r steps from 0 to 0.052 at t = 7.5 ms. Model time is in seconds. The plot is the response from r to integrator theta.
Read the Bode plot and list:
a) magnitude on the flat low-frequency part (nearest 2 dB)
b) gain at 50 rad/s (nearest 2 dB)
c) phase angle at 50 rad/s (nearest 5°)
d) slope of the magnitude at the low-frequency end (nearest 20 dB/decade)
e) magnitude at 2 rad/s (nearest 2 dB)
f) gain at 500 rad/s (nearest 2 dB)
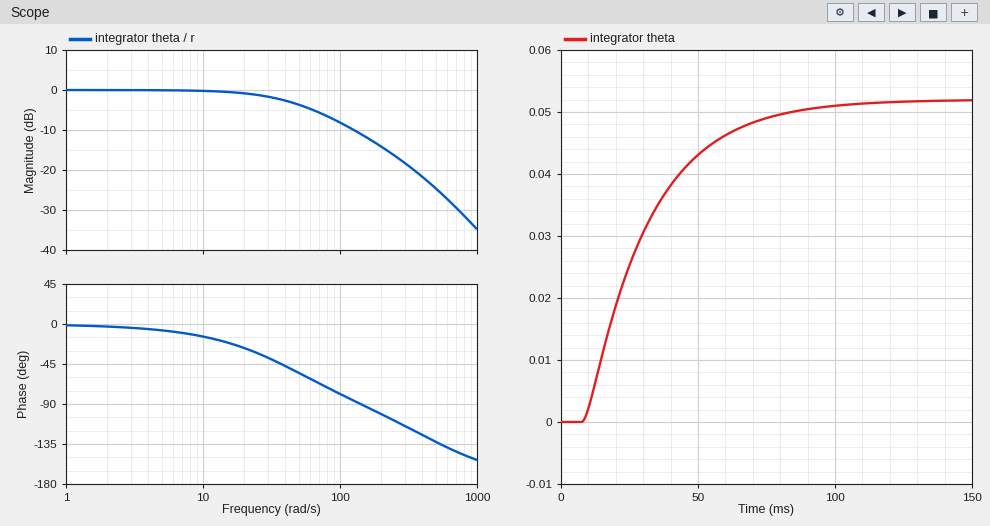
0 dB
-4 dB
-55°
0 dB/decade
0 dB
-24 dB
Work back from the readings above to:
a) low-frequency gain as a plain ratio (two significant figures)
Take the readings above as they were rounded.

1.0
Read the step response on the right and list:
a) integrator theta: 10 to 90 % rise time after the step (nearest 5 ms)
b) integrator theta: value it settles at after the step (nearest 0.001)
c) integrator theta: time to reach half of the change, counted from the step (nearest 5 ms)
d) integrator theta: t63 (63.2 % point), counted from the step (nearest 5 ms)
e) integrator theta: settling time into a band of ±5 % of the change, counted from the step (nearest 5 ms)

50 ms
0.052
20 ms
25 ms
70 ms
